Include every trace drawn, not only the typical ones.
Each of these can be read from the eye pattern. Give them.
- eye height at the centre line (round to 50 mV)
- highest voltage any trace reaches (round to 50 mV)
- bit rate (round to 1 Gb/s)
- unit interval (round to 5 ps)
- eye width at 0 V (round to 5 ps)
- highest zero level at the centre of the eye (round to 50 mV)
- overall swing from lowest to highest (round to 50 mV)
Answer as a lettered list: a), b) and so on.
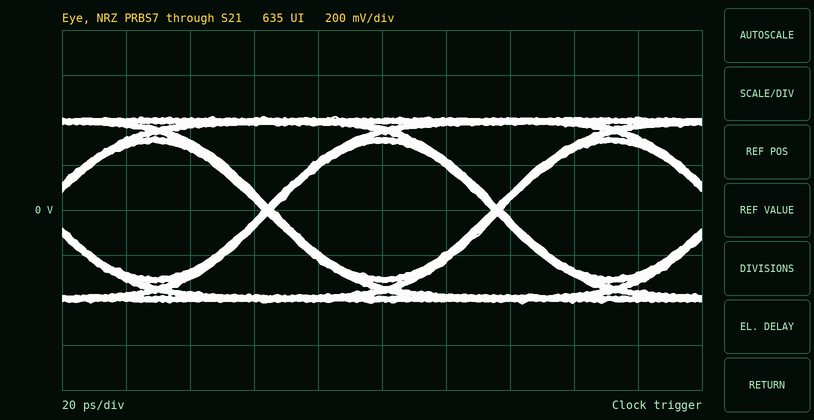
a) 600 mV
b) 400 mV
c) 14 Gb/s
d) 70 ps
e) 70 ps
f) -300 mV
g) 850 mV
